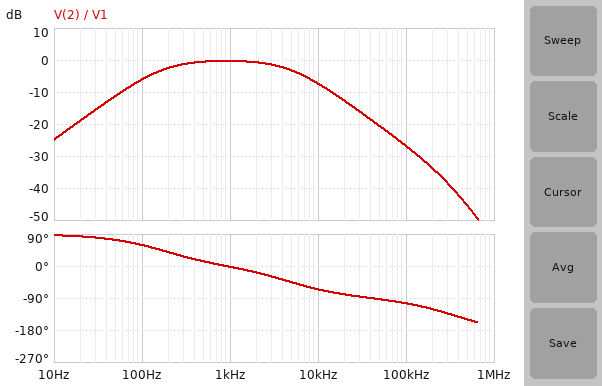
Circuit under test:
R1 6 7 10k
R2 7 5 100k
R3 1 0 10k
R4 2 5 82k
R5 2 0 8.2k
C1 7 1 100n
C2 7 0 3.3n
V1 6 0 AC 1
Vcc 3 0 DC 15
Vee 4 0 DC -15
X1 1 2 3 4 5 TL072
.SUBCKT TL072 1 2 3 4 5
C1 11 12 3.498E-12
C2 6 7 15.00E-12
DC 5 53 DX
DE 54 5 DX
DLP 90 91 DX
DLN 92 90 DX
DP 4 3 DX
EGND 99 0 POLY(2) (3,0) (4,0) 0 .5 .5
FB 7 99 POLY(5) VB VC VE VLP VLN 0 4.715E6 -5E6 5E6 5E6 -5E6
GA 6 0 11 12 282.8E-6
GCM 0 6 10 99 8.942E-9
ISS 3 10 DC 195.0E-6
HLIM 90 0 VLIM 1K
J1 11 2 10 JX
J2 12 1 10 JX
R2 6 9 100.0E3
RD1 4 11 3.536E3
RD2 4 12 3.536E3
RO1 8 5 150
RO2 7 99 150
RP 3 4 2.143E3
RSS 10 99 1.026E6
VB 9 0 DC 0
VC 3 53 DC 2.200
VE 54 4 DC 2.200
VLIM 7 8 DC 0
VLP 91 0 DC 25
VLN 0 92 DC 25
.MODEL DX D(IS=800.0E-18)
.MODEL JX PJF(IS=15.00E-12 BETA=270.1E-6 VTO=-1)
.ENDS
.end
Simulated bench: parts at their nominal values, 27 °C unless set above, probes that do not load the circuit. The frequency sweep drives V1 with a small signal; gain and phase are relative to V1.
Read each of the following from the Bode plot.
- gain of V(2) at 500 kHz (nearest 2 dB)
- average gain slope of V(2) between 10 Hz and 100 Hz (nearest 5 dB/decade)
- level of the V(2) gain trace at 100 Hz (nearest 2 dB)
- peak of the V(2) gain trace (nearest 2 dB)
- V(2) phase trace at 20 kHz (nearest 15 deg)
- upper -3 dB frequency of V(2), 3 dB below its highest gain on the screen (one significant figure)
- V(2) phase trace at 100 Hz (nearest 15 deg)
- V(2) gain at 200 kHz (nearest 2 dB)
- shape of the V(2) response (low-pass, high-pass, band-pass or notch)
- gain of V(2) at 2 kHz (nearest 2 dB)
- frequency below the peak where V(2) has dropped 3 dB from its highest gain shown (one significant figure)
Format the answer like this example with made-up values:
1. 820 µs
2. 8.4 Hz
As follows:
1. -46 dB
2. 20 dB/decade
3. -6 dB
4. 0 dB
5. -75 deg
6. 5 kHz
7. 60 deg
8. -34 dB
9. band-pass
10. 0 dB
11. 200 Hz
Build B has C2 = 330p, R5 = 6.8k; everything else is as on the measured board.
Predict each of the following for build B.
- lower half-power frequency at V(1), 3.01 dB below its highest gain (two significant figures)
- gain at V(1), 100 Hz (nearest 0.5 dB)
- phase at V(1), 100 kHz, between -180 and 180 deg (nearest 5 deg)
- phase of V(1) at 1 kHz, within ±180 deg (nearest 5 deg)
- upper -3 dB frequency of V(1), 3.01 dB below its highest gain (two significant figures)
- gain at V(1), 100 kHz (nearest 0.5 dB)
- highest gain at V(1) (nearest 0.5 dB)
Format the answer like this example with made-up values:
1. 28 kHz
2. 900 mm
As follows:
1. 220 Hz
2. -5.5 dB
3. -70 deg
4. 10 deg
5. 31 kHz
6. -8.5 dB
7. 2.0 dB
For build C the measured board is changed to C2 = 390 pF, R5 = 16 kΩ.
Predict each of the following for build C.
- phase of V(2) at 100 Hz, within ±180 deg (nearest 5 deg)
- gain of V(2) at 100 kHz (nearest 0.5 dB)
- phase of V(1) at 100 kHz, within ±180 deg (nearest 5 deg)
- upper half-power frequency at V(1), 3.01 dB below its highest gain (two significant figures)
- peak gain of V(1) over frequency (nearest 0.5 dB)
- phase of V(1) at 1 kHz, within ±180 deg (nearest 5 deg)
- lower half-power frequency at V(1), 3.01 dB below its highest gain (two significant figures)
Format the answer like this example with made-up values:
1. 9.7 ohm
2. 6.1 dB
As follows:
1. 50 deg
2. -9.5 dB
3. -60 deg
4. 58 kHz
5. -3.5 dB
6. 5 deg
7. 120 Hz
